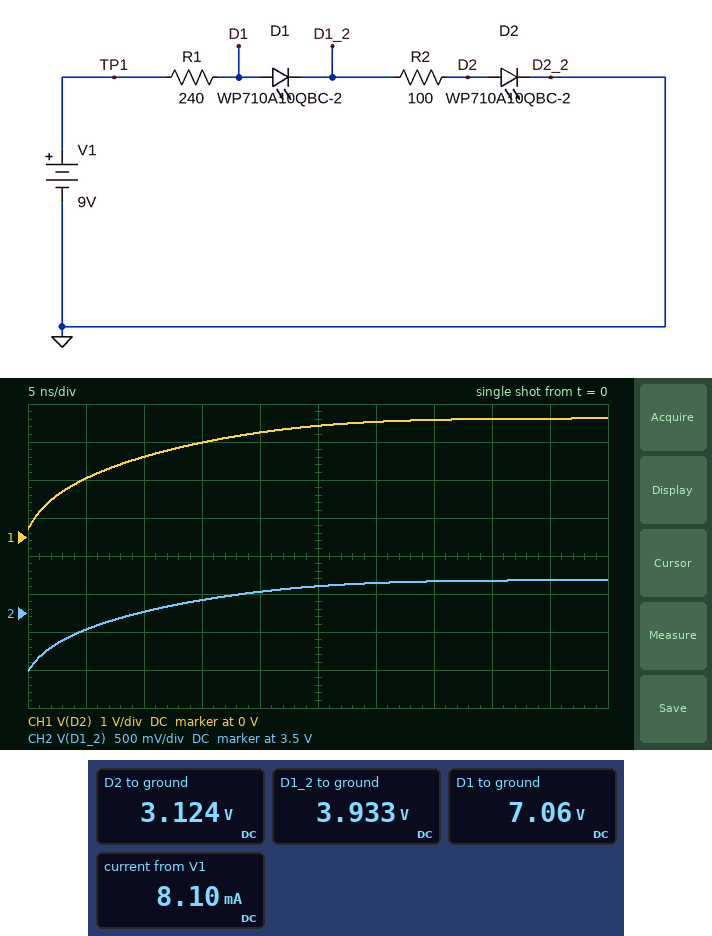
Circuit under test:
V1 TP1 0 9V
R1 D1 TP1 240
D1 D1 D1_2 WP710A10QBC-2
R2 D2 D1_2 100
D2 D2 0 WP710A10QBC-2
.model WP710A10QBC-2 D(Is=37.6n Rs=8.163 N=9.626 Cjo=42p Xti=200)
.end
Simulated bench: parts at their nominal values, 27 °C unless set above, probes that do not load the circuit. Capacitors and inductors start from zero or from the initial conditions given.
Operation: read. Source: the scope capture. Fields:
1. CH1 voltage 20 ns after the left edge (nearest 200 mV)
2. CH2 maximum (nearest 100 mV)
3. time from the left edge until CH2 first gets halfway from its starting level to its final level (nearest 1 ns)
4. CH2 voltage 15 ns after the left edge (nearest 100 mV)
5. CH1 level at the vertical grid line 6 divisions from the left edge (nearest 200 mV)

2.8 V
3.9 V
6 ns
3.7 V
3.0 V
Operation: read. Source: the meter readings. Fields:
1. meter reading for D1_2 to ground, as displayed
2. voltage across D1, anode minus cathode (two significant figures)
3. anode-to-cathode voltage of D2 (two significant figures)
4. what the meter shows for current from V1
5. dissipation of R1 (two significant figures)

3.933 V
3.1 V
3.1 V
8.10 mA
16 mW
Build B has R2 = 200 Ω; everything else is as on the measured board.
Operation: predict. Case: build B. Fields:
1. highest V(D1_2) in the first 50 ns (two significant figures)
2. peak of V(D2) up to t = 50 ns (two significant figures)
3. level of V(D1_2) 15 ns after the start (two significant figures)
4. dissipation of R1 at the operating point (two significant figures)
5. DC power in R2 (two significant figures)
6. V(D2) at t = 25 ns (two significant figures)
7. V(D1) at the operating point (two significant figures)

4.4 V
3.0 V
4.3 V
10 mW
8.6 mW
2.7 V
7.4 V
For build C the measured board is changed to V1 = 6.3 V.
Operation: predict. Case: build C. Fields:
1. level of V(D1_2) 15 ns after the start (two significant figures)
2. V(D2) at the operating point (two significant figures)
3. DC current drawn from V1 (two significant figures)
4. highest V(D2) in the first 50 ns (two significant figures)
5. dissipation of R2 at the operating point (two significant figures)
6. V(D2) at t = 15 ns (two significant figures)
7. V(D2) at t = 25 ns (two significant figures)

2.6 V
2.8 V
2.3 mA
2.7 V
520 µW
1.9 V
2.3 V
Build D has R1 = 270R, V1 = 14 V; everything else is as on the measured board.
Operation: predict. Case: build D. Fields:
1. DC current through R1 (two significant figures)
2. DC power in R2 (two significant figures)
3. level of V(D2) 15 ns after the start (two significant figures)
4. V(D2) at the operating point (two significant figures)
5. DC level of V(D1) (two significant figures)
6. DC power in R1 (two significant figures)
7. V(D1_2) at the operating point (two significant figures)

19 mA
37 mW
3.2 V
3.4 V
8.8 V
100 mW
5.4 V
